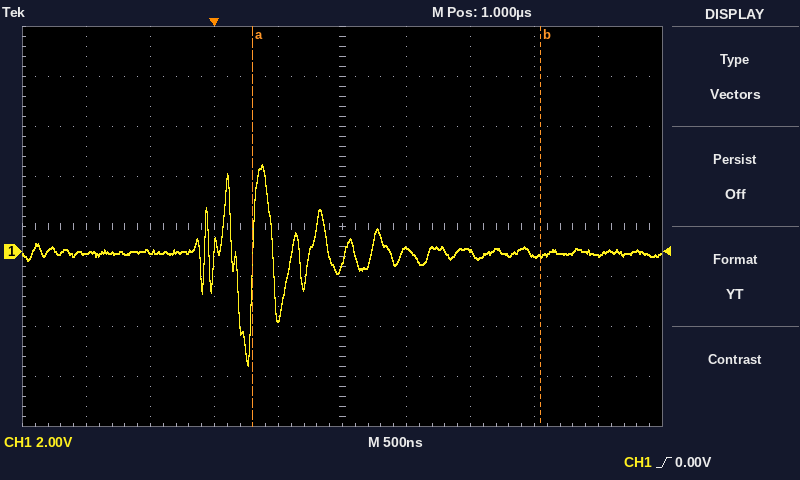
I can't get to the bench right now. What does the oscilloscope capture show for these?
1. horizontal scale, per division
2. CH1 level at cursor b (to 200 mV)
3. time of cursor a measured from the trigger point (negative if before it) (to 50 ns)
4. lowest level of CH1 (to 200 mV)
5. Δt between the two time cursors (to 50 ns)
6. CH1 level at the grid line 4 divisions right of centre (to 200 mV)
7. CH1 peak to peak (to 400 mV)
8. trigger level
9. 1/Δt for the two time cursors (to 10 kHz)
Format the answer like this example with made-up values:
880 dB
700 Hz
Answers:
500 ns
-200 mV
+300 ns
-4.6 V
2.25 µs
-200 mV
8.0 V
0.00 V
440 kHz
